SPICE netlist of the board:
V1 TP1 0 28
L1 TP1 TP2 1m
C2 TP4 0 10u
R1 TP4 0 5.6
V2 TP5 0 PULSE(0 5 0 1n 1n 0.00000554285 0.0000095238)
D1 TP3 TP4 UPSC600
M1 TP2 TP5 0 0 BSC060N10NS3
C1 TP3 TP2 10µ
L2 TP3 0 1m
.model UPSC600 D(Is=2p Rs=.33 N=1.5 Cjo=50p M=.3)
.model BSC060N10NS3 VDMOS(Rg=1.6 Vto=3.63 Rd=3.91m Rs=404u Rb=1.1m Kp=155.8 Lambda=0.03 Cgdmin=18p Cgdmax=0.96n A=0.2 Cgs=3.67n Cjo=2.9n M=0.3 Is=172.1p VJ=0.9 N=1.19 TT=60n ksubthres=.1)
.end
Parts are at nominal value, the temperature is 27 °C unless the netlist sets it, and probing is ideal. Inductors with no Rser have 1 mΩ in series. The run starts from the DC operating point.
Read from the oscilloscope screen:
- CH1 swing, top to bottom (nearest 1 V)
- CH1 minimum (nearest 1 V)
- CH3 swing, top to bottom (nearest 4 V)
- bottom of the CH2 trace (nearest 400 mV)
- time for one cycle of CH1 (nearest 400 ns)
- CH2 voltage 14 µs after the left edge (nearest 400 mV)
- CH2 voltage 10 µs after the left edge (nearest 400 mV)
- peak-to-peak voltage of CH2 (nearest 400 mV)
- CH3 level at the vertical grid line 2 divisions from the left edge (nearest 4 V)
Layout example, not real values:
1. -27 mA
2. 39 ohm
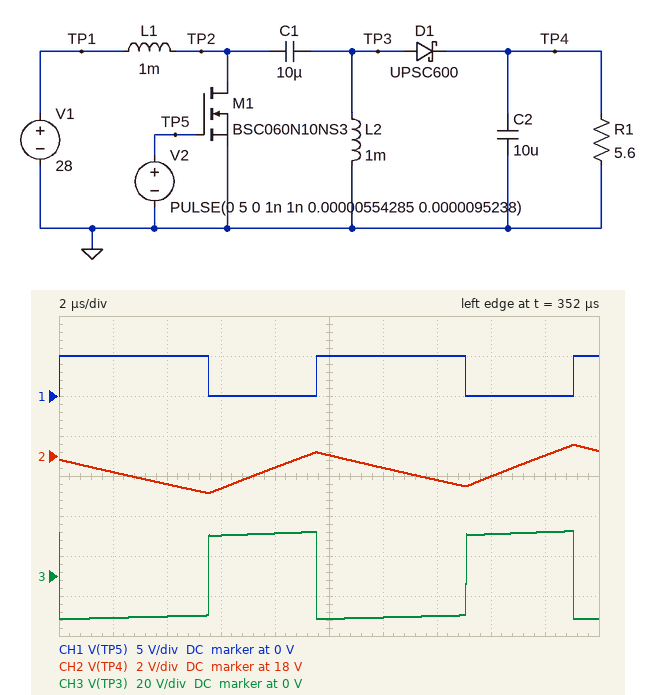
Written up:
1. 5 V
2. 0 V
3. 44 V
4. 16.0 V
5. 9.6 µs
6. 16.8 V
7. 18.0 V
8. 2.4 V
9. -20 V
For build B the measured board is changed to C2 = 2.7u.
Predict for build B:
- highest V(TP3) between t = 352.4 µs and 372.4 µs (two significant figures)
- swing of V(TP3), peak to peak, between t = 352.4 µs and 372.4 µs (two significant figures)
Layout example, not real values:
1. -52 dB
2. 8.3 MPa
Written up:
1. 25 V
2. 47 V
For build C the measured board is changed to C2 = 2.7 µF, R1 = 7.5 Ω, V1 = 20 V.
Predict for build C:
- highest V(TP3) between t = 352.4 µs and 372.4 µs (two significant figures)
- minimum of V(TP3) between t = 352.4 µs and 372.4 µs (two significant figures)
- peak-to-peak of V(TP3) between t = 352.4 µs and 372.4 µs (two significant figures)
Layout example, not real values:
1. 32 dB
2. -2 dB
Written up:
1. 21 V
2. -16 V
3. 37 V
